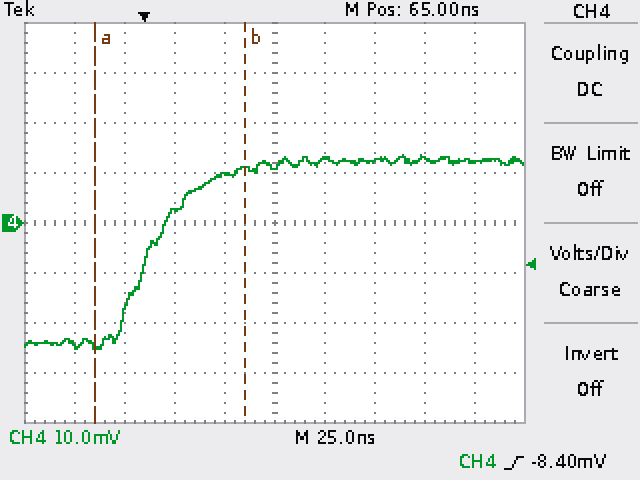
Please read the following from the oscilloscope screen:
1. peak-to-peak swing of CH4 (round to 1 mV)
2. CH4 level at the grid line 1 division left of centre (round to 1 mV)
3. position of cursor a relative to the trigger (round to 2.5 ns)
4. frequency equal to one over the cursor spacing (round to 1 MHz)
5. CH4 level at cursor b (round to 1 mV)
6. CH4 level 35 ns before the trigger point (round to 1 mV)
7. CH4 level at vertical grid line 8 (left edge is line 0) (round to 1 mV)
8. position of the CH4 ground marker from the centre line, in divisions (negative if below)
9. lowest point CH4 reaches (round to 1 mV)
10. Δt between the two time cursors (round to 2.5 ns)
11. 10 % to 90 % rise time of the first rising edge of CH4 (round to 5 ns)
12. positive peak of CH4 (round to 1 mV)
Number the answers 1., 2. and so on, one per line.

1. 39 mV
2. 10 mV
3. -25.0 ns
4. 13 MHz
5. 11 mV
6. -24 mV
7. 13 mV
8. 0.0 div
9. -25 mV
10. 75.0 ns
11. 45 ns
12. 14 mV
